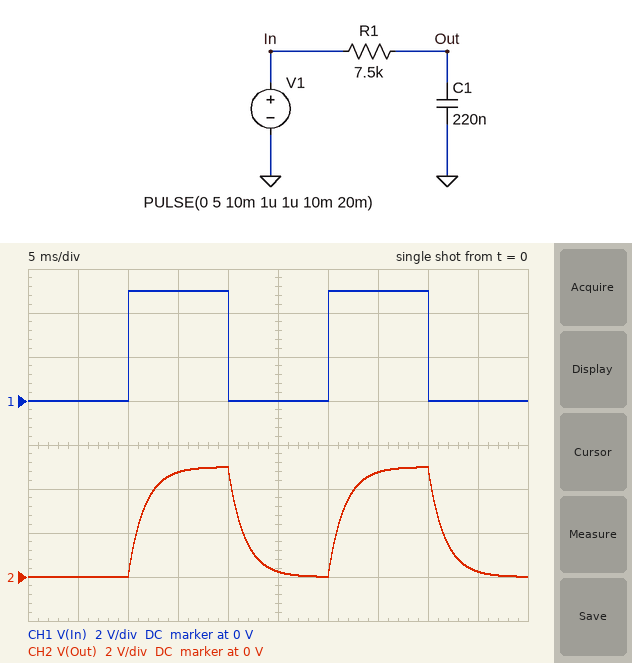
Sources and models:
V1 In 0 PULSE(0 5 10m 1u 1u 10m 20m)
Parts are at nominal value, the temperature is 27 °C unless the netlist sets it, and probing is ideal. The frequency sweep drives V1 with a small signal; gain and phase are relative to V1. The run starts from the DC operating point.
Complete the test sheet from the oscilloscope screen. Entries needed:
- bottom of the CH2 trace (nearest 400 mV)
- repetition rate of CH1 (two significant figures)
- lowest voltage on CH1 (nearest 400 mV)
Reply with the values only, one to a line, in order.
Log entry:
0 V
50 Hz
0 V
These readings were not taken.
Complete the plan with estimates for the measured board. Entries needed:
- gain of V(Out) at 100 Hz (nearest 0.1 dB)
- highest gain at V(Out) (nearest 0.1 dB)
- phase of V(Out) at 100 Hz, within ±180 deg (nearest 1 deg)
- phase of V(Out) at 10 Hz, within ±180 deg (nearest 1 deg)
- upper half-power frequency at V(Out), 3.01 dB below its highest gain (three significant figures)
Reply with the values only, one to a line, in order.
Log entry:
-3.2 dB
0 dB
-46 deg
-6 deg
96.5 Hz
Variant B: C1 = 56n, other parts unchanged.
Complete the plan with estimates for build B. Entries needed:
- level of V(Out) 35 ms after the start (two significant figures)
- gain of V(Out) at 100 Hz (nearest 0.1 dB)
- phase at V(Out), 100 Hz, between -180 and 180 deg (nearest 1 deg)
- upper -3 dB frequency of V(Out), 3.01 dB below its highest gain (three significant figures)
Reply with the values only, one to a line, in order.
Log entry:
5.0 V
-0.3 dB
-15 deg
379 Hz
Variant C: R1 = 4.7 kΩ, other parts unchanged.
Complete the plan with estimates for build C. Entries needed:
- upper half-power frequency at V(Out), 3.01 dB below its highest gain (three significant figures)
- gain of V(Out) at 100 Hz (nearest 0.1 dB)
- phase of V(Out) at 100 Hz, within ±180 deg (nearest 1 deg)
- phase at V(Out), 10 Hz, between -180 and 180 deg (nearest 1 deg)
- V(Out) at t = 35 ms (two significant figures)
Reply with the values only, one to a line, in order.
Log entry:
154 Hz
-1.5 dB
-33 deg
-4 deg
5.0 V
